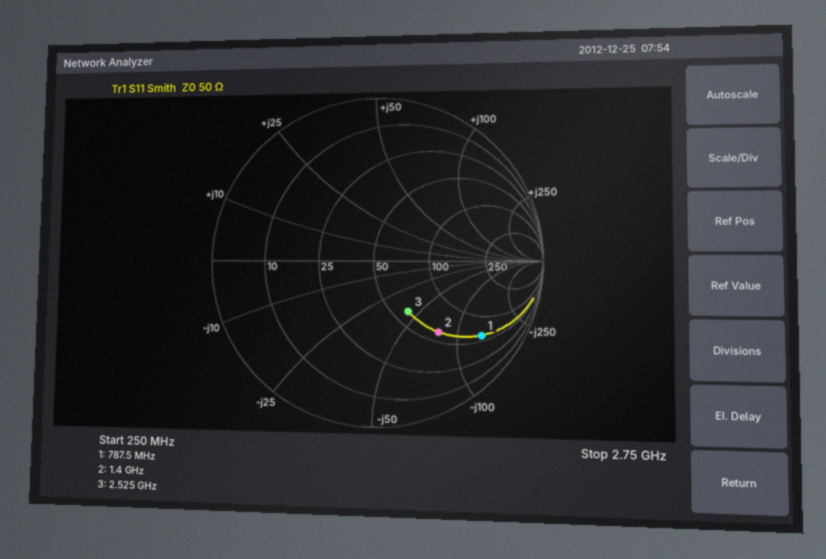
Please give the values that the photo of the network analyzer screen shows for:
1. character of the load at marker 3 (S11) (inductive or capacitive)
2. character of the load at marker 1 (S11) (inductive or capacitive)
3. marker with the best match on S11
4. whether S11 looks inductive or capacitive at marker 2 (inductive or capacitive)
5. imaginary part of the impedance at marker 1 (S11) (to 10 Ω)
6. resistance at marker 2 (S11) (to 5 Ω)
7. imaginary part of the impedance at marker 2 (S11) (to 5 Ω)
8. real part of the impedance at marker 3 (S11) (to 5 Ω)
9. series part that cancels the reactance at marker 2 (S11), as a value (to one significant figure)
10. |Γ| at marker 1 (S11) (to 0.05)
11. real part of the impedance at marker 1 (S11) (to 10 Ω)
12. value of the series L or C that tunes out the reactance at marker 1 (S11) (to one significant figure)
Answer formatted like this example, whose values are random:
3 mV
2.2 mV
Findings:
capacitive
capacitive
marker 3
capacitive
-140 Ω
60 Ω
-75 Ω
60 Ω
9 nH
0.80
60 Ω
30 nH
